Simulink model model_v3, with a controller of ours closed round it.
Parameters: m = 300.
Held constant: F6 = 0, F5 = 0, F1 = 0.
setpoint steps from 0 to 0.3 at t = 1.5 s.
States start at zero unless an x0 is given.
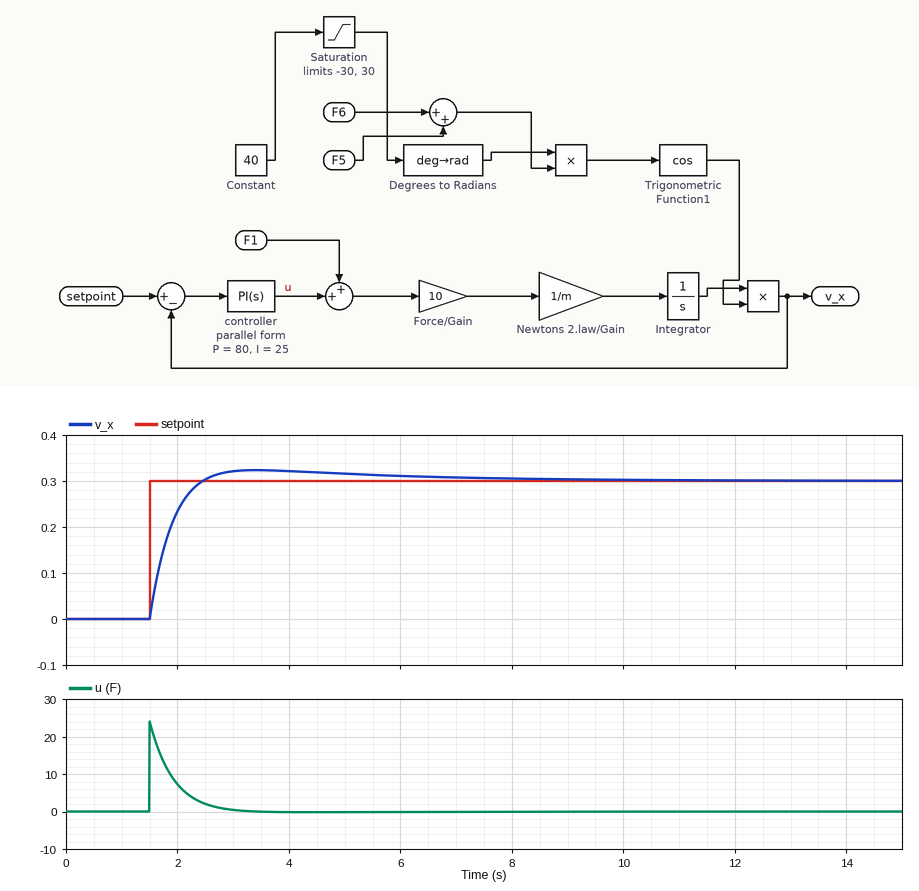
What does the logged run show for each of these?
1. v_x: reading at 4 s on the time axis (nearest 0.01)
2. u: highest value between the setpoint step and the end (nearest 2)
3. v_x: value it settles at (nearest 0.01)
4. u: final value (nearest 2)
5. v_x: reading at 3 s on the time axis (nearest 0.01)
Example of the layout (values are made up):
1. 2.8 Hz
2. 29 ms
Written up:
1. 0.32
2. 24
3. 0.30
4. 0
5. 0.32
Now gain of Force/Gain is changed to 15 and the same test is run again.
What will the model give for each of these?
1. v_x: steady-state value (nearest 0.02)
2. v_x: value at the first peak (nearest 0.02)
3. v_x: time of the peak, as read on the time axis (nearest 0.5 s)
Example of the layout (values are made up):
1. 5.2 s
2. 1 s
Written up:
1. 0.30
2. 0.32
3. 3.0 s
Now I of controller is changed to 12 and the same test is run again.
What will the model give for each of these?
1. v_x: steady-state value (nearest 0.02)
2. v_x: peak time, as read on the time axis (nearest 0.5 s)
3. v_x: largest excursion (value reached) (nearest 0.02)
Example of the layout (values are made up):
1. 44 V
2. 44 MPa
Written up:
1. 0.30
2. 4.0 s
3. 0.32
